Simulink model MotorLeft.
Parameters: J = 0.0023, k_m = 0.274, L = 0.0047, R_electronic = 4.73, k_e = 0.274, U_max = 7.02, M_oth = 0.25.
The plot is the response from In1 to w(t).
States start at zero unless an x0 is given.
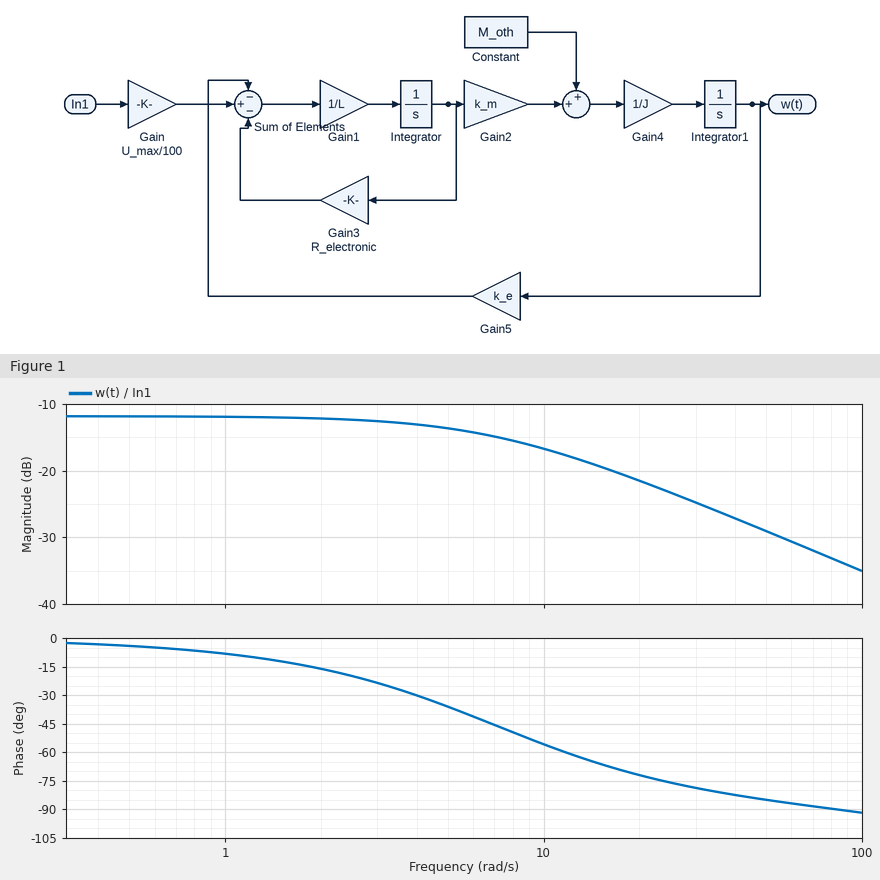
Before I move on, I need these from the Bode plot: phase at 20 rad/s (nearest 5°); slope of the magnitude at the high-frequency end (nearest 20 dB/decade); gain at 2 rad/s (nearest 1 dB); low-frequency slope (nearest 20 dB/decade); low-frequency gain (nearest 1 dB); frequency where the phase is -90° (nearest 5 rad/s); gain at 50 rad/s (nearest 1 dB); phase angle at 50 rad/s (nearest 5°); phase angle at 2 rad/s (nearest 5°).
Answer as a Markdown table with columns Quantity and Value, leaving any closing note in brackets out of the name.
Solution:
| Quantity | Value |
|---|---|
| phase at 20 rad/s | -70° |
| slope of the magnitude at the high-frequency end | -20 dB/decade |
| gain at 2 rad/s | -12 dB |
| low-frequency slope | 0 dB/decade |
| low-frequency gain | -12 dB |
| frequency where the phase is -90° | 85 rad/s |
| gain at 50 rad/s | -29 dB |
| phase angle at 50 rad/s | -85° |
| phase angle at 2 rad/s | -15° |
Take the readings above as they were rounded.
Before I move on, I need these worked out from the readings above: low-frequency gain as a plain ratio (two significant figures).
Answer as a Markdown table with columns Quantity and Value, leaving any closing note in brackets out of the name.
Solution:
| Quantity | Value |
|---|---|
| low-frequency gain as a plain ratio | 0.25 |
